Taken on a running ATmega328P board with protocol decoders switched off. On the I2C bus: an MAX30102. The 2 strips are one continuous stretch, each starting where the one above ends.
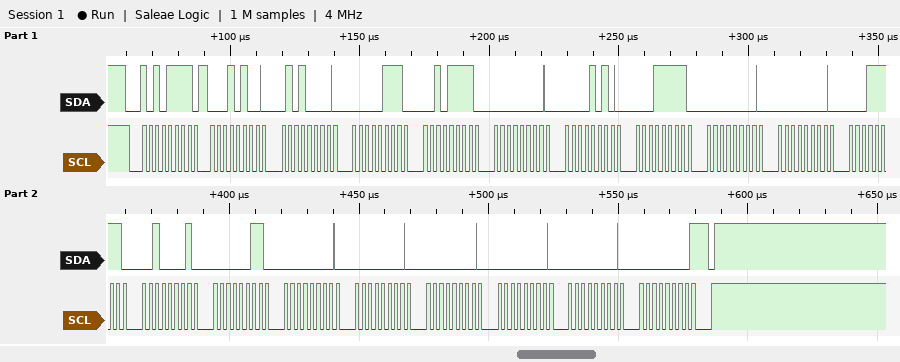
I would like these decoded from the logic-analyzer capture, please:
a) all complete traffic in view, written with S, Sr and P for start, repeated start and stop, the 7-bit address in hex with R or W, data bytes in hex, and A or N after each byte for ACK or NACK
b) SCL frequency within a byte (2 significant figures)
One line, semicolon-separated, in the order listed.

S 57R A 14 A 50 A 07 A 2F A 00 A 0A A 1F A 00 A 00 A 1F A 21 A 03 A 00 A 00 A 00 A 00 A 00 A 00 N P; 400 kHz
